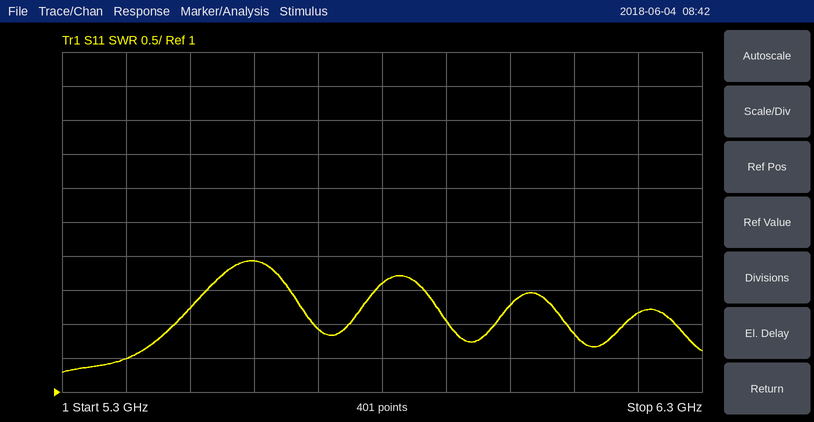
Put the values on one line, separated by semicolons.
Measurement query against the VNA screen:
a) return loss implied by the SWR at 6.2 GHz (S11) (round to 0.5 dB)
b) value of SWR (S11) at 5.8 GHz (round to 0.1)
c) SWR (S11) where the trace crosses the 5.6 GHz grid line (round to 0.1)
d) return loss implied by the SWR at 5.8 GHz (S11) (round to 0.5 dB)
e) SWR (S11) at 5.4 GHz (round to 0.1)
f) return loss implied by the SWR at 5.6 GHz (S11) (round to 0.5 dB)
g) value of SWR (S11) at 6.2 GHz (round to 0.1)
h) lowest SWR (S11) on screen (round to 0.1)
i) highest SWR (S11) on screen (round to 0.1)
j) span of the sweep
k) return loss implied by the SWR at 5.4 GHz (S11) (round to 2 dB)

8.5 dB; 2.6; 2.9; 7.0 dB; 1.5; 6.0 dB; 2.2; 1.3; 2.9; 1 GHz; 14 dB
